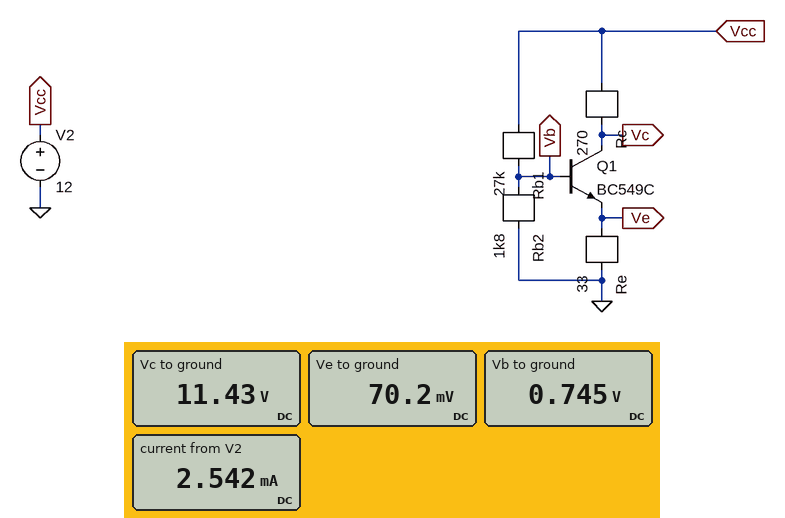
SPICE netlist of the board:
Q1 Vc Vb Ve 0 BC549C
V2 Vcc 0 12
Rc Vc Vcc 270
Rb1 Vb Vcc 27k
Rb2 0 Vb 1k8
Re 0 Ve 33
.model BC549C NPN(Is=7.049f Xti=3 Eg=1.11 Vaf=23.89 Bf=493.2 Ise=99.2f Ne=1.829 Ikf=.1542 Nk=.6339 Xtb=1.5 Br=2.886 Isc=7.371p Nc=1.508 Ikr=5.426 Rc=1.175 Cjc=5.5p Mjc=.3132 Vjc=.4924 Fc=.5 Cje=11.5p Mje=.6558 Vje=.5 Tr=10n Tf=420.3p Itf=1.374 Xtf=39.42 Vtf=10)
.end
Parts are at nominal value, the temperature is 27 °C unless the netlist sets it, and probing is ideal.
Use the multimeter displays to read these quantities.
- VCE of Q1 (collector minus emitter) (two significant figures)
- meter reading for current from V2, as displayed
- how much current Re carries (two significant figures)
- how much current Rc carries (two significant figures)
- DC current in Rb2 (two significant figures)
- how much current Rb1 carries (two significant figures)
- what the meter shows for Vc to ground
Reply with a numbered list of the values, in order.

1. 11 V
2. 2.542 mA
3. 2.1 mA
4. 2.1 mA
5. 410 µA
6. 420 µA
7. 11.43 V
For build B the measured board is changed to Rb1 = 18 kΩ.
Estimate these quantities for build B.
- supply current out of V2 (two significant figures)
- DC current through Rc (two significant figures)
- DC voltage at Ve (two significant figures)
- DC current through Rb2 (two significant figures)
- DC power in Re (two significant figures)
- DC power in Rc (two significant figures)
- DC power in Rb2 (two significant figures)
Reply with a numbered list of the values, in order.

1. 11 mA
2. 10 mA
3. 340 mV
4. 590 µA
5. 3.6 mW
6. 29 mW
7. 630 µW
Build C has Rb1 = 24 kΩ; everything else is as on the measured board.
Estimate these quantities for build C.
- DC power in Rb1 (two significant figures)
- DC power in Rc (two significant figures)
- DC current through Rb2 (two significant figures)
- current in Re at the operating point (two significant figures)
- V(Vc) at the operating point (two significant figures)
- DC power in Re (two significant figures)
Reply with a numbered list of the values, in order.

1. 5.2 mW
2. 4.5 mW
3. 460 µA
4. 4.1 mA
5. 11 V
6. 550 µW
